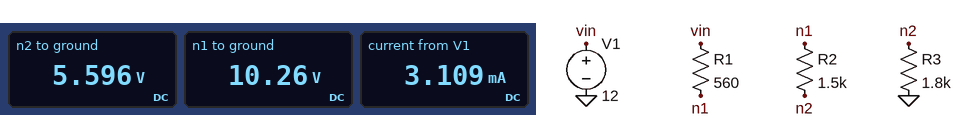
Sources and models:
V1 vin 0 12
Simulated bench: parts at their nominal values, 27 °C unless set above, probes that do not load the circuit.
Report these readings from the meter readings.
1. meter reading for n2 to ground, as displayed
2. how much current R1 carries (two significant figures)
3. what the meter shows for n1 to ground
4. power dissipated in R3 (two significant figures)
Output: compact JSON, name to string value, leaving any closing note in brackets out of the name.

{"meter reading for n2 to ground, as displayed": "5.596 V", "how much current R1 carries": "3.1 mA", "what the meter shows for n1 to ground": "10.26 V", "power dissipated in R3": "17 mW"}
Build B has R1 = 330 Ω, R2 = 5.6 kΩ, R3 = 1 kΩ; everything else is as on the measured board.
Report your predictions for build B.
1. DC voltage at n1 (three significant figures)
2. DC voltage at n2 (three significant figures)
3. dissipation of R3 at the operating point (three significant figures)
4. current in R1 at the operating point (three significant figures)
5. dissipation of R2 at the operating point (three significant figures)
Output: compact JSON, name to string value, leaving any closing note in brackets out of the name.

{"DC voltage at n1": "11.4 V", "DC voltage at n2": "1.73 V", "dissipation of R3 at the operating point": "3.00 mW", "current in R1 at the operating point": "1.73 mA", "dissipation of R2 at the operating point": "16.8 mW"}
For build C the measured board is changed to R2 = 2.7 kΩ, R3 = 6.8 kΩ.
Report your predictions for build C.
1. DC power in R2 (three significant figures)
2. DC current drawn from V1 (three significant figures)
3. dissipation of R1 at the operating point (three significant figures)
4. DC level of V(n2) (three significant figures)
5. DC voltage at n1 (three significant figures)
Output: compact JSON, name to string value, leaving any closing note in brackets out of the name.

{"DC power in R2": "3.84 mW", "DC current drawn from V1": "1.19 mA", "dissipation of R1 at the operating point": "797 µW", "DC level of V(n2)": "8.11 V", "DC voltage at n1": "11.3 V"}
